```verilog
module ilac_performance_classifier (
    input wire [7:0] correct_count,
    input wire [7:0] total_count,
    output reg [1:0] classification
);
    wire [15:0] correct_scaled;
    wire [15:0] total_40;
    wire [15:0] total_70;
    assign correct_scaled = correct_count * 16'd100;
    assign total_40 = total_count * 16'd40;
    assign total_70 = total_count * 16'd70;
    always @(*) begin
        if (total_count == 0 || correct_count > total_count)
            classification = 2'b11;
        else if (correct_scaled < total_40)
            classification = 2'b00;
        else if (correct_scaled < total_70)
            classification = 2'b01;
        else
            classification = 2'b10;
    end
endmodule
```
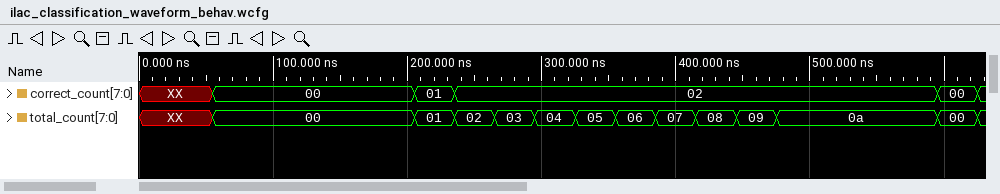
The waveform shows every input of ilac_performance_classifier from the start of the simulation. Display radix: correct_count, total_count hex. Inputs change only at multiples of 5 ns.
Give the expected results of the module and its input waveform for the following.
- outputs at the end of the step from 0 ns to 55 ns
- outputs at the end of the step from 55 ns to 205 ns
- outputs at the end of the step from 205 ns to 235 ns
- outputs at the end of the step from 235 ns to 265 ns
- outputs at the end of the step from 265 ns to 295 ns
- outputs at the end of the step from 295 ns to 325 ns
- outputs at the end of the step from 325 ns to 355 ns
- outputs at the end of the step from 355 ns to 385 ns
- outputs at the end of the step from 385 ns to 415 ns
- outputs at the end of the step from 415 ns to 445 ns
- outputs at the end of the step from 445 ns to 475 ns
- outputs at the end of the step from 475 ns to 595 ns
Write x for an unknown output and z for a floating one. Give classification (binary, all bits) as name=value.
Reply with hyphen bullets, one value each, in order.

- classification=x
- classification=11
- classification=10
- classification=10
- classification=01
- classification=01
- classification=01
- classification=00
- classification=00
- classification=00
- classification=00
- classification=00
